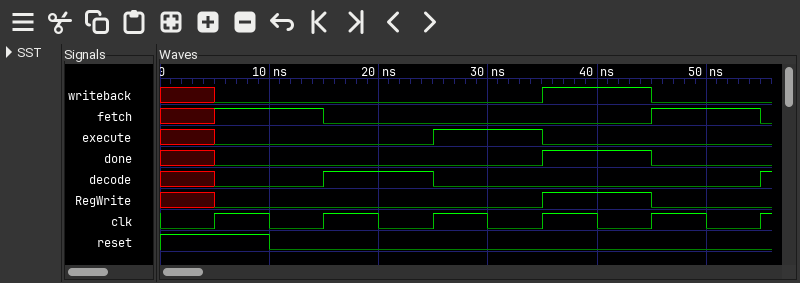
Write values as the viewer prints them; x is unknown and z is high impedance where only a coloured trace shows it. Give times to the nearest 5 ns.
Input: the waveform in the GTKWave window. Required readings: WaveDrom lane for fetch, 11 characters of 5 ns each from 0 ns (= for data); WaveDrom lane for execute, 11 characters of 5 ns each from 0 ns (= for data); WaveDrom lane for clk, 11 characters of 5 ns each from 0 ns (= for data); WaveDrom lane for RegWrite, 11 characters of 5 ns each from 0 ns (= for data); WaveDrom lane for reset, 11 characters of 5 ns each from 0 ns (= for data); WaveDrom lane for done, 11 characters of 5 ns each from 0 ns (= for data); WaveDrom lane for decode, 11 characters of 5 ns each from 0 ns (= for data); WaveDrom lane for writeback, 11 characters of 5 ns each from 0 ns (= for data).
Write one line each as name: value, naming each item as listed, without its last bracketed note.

WaveDrom lane for fetch, 11 characters of 5 ns each from 0 ns: {name: 'fetch', wave: 'x1.0.....1.'}
WaveDrom lane for execute, 11 characters of 5 ns each from 0 ns: {name: 'execute', wave: 'x0...1.0...'}
WaveDrom lane for clk, 11 characters of 5 ns each from 0 ns: {name: 'clk', wave: '01010101010'}
WaveDrom lane for RegWrite, 11 characters of 5 ns each from 0 ns: {name: 'RegWrite', wave: 'x0.....1.0.'}
WaveDrom lane for reset, 11 characters of 5 ns each from 0 ns: {name: 'reset', wave: '1.0........'}
WaveDrom lane for done, 11 characters of 5 ns each from 0 ns: {name: 'done', wave: 'x0.....1.0.'}
WaveDrom lane for decode, 11 characters of 5 ns each from 0 ns: {name: 'decode', wave: 'x0.1.0.....'}
WaveDrom lane for writeback, 11 characters of 5 ns each from 0 ns: {name: 'writeback', wave: 'x0.....1.0.'}
